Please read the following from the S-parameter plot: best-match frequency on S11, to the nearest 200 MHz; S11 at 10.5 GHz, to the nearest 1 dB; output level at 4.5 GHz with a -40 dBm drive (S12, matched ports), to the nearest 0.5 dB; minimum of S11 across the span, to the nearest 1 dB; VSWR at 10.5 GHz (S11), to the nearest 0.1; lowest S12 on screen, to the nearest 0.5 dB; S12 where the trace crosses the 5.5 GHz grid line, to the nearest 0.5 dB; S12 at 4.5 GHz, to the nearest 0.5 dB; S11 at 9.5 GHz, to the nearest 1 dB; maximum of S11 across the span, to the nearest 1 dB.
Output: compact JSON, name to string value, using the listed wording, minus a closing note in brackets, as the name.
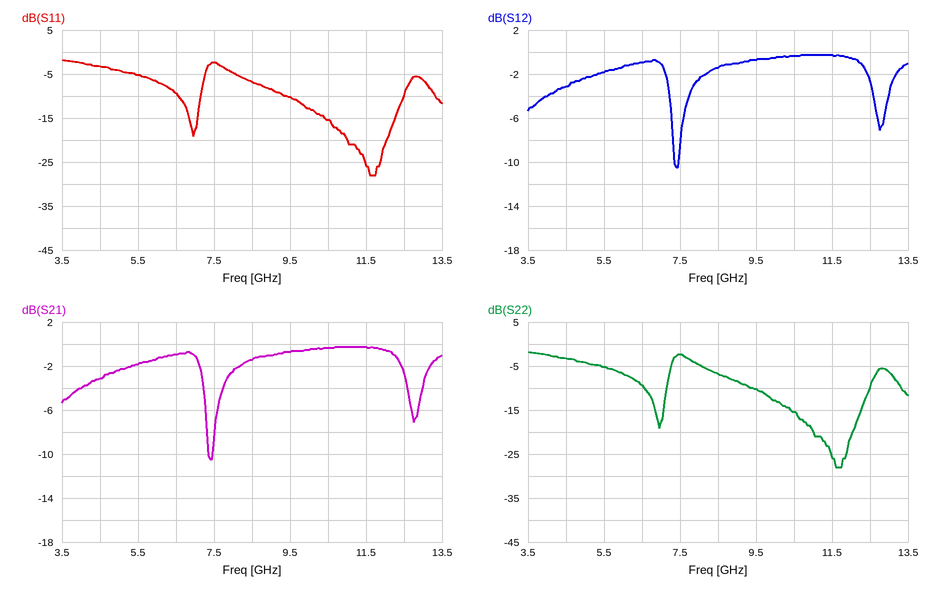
{"best-match frequency on S11, to the nearest 200 MHz": "11.6 GHz", "S11 at 10.5 GHz, to the nearest 1 dB": "-15 dB", "output level at 4.5 GHz with a -40 dBm drive (S12, matched ports), to the nearest 0.5 dB": "-43.0 dBm", "minimum of S11 across the span, to the nearest 1 dB": "-28 dB", "VSWR at 10.5 GHz (S11), to the nearest 0.1": "1.4", "lowest S12 on screen, to the nearest 0.5 dB": "-10.5 dB", "S12 where the trace crosses the 5.5 GHz grid line, to the nearest 0.5 dB": "-2.0 dB", "S12 at 4.5 GHz, to the nearest 0.5 dB": "-3.0 dB", "S11 at 9.5 GHz, to the nearest 1 dB": "-10 dB", "maximum of S11 across the span, to the nearest 1 dB": "-2 dB"}
